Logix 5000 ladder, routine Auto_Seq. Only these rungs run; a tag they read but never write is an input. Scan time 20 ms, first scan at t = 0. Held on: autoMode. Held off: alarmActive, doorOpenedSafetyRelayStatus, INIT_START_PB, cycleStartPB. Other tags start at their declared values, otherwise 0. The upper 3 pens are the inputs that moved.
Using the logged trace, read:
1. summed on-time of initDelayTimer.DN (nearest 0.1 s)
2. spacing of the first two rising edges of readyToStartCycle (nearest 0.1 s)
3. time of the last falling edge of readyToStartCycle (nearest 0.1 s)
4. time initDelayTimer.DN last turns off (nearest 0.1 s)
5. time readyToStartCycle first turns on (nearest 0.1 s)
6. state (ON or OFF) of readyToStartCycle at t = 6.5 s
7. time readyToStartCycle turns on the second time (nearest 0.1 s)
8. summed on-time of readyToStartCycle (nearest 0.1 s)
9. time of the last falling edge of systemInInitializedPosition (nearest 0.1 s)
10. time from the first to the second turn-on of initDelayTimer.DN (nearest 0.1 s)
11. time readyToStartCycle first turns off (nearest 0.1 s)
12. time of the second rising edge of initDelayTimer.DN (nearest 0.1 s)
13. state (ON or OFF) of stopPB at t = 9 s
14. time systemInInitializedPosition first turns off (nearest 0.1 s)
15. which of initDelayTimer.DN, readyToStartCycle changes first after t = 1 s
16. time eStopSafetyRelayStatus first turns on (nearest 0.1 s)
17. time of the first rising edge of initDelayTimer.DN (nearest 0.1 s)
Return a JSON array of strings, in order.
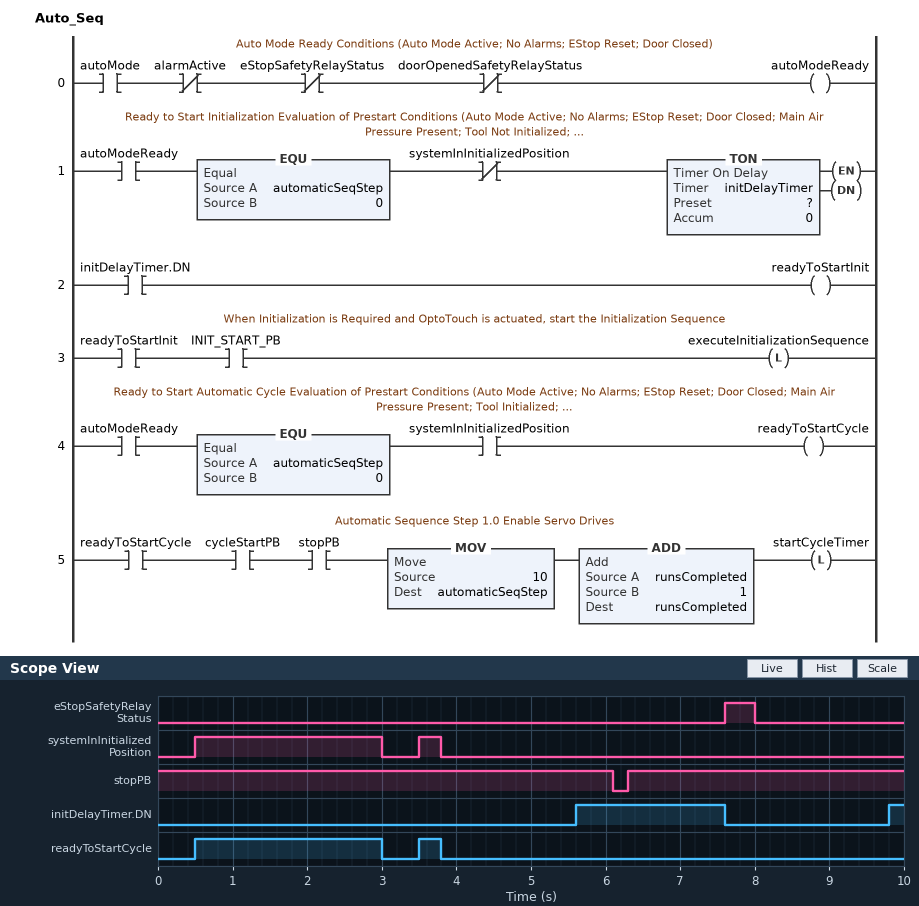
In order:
["2.2 s", "3.0 s", "3.8 s", "7.6 s", "0.5 s", "OFF", "3.5 s", "2.8 s", "3.8 s", "4.2 s", "3.0 s", "9.8 s", "ON", "3.0 s", "readyToStartCycle", "7.6 s", "5.6 s"]
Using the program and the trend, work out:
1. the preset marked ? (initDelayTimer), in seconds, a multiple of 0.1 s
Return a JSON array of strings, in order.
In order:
["1.8 s"]
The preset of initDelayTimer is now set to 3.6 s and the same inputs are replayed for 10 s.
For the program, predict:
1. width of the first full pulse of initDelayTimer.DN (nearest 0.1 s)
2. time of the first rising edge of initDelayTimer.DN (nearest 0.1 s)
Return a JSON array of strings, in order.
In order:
["0.2 s", "7.4 s"]
